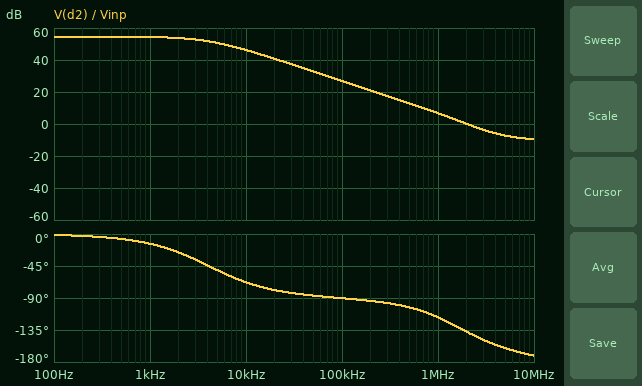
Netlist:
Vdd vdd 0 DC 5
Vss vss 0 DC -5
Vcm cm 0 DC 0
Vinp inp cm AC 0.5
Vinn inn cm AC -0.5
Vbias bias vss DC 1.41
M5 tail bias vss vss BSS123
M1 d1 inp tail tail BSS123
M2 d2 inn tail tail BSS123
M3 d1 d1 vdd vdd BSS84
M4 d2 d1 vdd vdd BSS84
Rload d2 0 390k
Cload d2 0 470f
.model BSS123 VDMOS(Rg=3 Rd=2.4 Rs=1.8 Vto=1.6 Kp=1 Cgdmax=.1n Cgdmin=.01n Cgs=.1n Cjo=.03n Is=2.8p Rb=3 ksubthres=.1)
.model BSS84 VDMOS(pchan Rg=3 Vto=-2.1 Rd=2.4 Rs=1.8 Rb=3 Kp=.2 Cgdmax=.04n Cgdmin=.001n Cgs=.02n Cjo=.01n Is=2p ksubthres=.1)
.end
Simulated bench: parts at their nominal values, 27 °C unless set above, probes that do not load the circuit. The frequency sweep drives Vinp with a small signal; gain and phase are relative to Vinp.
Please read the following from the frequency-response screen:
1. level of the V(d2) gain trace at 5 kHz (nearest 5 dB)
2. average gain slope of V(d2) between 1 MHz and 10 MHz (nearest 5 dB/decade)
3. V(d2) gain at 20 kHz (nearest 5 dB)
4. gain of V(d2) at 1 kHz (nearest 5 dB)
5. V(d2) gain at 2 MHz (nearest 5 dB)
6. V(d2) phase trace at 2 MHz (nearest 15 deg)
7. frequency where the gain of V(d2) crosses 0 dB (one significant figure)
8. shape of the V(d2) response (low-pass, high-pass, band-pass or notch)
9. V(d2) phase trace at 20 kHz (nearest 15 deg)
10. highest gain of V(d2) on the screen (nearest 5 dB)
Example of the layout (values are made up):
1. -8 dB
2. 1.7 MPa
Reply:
1. 50 dB
2. -15 dB/decade
3. 40 dB
4. 55 dB
5. 0 dB
6. -135 deg
7. 2 MHz
8. low-pass
9. -75 deg
10. 55 dB
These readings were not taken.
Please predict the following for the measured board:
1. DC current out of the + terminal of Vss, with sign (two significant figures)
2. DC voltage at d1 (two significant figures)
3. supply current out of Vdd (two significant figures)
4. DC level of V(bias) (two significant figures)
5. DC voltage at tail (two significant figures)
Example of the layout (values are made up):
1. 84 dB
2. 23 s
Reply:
1. -97 µA
2. 3.0 V
3. 97 µA
4. -3.6 V
5. -1.4 V
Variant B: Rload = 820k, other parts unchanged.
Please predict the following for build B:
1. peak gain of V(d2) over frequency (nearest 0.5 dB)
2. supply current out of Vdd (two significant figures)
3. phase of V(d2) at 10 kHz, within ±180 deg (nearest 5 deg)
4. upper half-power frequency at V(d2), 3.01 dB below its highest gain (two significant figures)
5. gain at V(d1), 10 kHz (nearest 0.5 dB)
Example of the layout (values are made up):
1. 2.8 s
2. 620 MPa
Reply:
1. 61.0 dB
2. 97 µA
3. -80 deg
4. 2.0 kHz
5. -5.0 dB
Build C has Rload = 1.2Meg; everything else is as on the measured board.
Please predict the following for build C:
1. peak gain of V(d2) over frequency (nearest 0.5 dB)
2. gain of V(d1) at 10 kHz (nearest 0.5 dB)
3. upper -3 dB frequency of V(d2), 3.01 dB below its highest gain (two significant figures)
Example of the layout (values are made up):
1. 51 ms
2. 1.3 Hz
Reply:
1. 64.5 dB
2. -5.0 dB
3. 1.3 kHz
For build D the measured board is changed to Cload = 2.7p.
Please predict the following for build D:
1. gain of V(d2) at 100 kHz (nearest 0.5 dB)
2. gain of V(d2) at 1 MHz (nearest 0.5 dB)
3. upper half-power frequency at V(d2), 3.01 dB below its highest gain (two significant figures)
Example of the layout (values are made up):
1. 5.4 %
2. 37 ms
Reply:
1. 26.5 dB
2. 6.5 dB
3. 4.0 kHz
